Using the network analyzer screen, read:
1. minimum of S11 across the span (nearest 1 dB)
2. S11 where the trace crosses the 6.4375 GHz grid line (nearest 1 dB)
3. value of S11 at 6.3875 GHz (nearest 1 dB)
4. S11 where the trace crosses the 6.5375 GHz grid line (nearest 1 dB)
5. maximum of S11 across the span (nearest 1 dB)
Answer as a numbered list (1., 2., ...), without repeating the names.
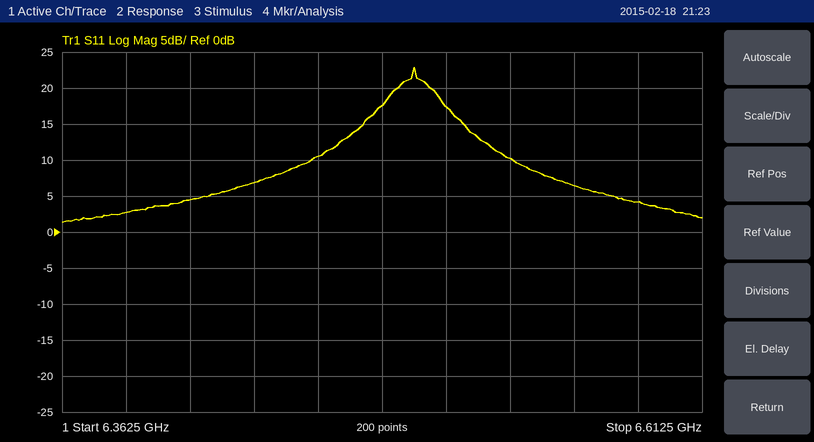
1. 1 dB
2. 7 dB
3. 3 dB
4. 10 dB
5. 23 dB
